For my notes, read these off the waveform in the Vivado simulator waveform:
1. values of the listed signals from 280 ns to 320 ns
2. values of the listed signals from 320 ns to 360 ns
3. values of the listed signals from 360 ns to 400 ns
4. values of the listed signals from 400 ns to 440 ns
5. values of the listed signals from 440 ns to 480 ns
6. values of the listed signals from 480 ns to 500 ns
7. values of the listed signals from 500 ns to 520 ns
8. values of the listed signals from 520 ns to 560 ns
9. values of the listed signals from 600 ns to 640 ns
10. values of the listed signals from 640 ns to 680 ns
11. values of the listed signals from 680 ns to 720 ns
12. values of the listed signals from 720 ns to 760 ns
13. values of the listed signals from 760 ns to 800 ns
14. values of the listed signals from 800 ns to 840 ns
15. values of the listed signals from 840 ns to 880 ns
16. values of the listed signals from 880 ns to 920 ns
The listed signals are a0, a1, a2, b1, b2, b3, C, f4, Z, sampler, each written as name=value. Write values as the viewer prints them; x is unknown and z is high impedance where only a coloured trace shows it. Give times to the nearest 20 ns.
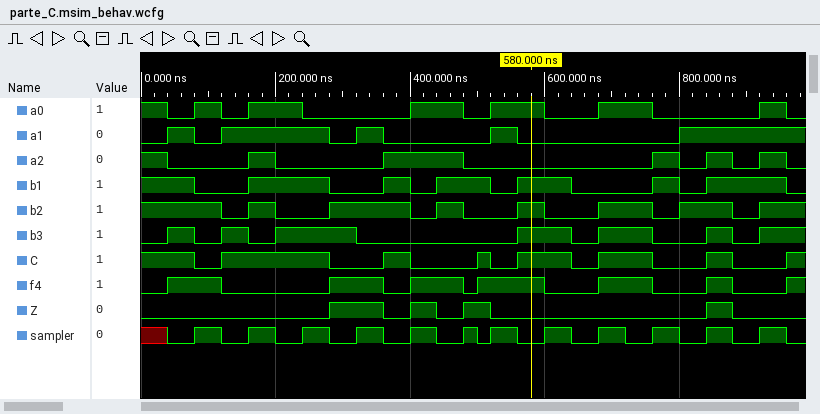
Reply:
a0=0, a1=0, a2=0, b1=0, b2=1, b3=1, C=0, f4=1, Z=1, sampler=0
a0=0, a1=1, a2=0, b1=0, b2=1, b3=0, C=0, f4=1, Z=1, sampler=1
a0=0, a1=0, a2=1, b1=1, b2=1, b3=0, C=1, f4=0, Z=0, sampler=0
a0=1, a1=0, a2=1, b1=0, b2=0, b3=0, C=0, f4=1, Z=1, sampler=1
a0=1, a1=0, a2=1, b1=1, b2=1, b3=0, C=0, f4=1, Z=0, sampler=0
a0=0, a1=0, a2=0, b1=1, b2=0, b3=0, C=0, f4=0, Z=1, sampler=1
a0=0, a1=0, a2=0, b1=1, b2=0, b3=0, C=1, f4=1, Z=1, sampler=0
a0=1, a1=1, a2=0, b1=0, b2=0, b3=0, C=0, f4=1, Z=0, sampler=1
a0=0, a1=0, a2=0, b1=1, b2=0, b3=1, C=1, f4=0, Z=0, sampler=1
a0=0, a1=0, a2=0, b1=0, b2=0, b3=0, C=0, f4=0, Z=0, sampler=0
a0=1, a1=0, a2=0, b1=0, b2=1, b3=1, C=1, f4=1, Z=0, sampler=1
a0=1, a1=0, a2=0, b1=0, b2=1, b3=1, C=1, f4=1, Z=0, sampler=0
a0=0, a1=0, a2=1, b1=1, b2=0, b3=0, C=0, f4=0, Z=0, sampler=1
a0=0, a1=1, a2=0, b1=0, b2=1, b3=0, C=0, f4=0, Z=0, sampler=0
a0=0, a1=1, a2=1, b1=1, b2=1, b3=1, C=1, f4=1, Z=1, sampler=1
a0=0, a1=1, a2=0, b1=1, b2=0, b3=0, C=0, f4=0, Z=0, sampler=0
